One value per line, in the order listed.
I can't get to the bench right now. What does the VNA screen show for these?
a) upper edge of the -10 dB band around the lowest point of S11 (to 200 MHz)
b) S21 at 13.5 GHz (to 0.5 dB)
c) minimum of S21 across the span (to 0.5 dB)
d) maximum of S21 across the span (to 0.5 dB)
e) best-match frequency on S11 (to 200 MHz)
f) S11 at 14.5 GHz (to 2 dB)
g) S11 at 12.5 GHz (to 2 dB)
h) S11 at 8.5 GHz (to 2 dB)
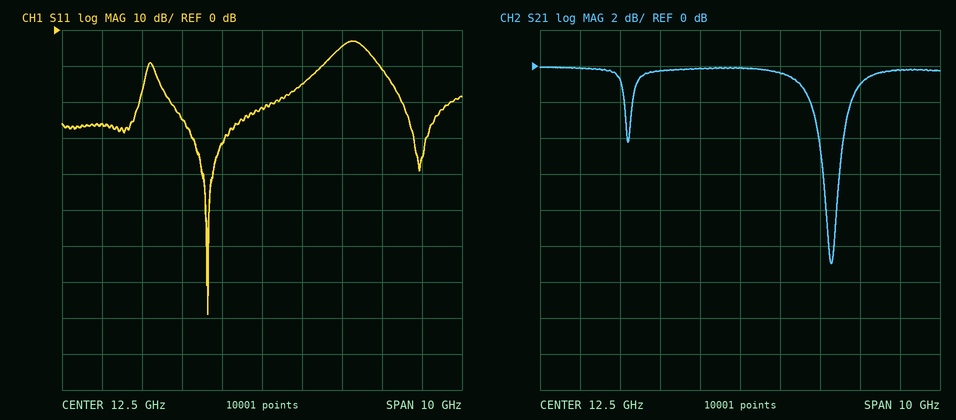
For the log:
14.0 GHz
-0.5 dB
-11.0 dB
0.0 dB
11.2 GHz
-4 dB
-22 dB
-26 dB
